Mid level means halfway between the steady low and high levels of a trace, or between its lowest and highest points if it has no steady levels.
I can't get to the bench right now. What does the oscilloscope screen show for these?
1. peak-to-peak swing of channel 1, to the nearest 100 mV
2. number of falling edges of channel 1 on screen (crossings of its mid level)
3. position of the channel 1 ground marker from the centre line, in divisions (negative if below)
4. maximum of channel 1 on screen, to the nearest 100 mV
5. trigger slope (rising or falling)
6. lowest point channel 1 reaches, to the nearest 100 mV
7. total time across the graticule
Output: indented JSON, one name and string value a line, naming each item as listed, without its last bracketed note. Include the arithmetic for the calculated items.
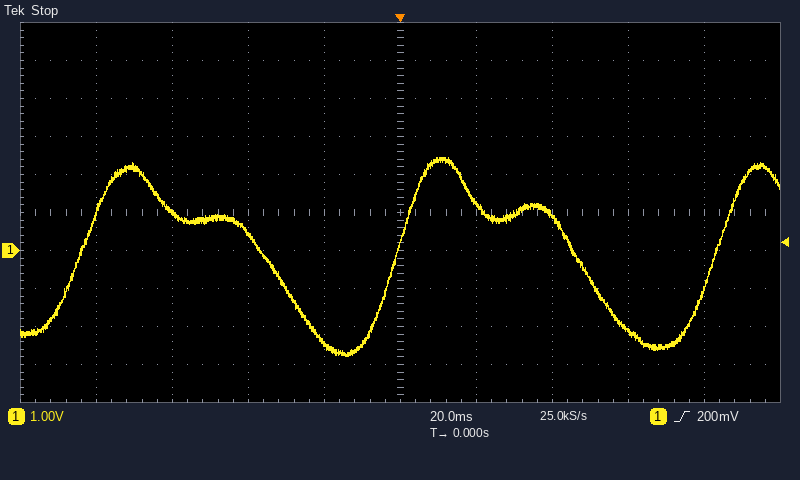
{
  "peak-to-peak swing of channel 1, to the nearest 100 mV": "2.4 V − (-2.8 V) = 5.2 V",
  "number of falling edges of channel 1 on screen": "2",
  "position of the channel 1 ground marker from the centre line, in divisions": "-1.0 div",
  "maximum of channel 1 on screen, to the nearest 100 mV": "2.4 V",
  "trigger slope": "rising",
  "lowest point channel 1 reaches, to the nearest 100 mV": "-2.8 V",
  "total time across the graticule": "200 ms"
}
